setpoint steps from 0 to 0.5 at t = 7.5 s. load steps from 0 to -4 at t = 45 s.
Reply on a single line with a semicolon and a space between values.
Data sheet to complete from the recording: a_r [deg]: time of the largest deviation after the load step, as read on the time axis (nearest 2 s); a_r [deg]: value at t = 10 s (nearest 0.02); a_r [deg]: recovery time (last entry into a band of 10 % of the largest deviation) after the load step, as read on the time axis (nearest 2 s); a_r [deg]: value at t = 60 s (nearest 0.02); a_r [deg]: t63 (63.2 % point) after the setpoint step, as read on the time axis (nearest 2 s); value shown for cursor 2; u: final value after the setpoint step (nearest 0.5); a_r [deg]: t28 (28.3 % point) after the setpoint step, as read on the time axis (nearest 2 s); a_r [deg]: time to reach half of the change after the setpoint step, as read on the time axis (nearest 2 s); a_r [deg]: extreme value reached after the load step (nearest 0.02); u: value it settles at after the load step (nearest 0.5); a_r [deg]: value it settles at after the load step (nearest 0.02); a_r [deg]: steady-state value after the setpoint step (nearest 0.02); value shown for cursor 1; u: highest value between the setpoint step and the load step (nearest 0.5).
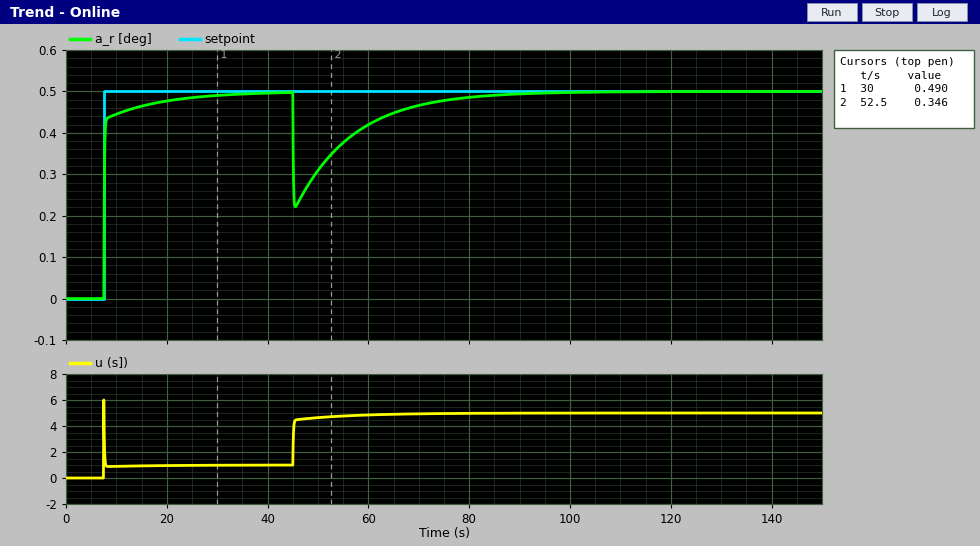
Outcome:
46 s; 0.44; 72 s; 0.42; 8 s; 0.346; 1.0; 8 s; 8 s; 0.22; 5.0; 0.50; 0.50; 0.490; 6.0
